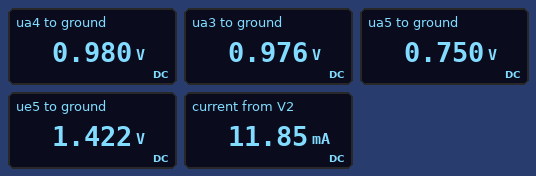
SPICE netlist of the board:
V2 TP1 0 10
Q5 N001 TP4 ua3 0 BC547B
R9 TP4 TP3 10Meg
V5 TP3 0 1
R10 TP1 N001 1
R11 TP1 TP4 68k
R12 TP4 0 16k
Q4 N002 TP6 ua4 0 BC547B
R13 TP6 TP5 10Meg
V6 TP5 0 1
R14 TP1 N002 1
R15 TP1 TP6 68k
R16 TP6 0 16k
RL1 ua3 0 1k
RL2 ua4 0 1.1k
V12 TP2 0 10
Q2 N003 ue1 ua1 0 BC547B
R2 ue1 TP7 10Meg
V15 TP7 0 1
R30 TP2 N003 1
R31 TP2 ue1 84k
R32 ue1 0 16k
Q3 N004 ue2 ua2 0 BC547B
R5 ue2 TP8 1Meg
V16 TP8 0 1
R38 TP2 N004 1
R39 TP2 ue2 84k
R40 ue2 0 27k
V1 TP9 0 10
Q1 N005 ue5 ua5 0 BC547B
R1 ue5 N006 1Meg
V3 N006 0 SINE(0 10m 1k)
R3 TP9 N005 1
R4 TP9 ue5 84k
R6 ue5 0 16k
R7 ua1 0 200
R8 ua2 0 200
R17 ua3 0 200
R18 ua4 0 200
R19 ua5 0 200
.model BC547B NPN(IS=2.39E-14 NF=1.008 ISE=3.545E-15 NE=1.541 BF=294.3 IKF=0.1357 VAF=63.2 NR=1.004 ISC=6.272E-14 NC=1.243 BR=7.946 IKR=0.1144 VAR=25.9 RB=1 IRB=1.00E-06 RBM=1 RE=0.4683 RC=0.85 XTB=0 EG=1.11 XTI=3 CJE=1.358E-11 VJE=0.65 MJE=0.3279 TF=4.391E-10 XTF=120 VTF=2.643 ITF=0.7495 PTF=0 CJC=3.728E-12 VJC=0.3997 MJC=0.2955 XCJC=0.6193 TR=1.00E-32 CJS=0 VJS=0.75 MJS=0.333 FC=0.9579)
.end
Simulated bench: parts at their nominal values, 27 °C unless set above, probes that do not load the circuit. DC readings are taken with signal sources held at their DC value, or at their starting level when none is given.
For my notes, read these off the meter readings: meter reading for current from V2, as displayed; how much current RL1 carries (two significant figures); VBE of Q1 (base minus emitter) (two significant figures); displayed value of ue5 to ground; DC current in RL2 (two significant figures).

11.85 mA
980 µA
670 mV
1.422 V
890 µA
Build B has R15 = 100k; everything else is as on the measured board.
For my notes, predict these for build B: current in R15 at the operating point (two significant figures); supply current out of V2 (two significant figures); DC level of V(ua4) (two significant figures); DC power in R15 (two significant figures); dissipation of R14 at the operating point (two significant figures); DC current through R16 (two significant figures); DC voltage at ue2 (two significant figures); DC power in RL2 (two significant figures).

88 µA
9.4 mA
570 mV
770 µW
11 µW
77 µA
2.0 V
290 µW
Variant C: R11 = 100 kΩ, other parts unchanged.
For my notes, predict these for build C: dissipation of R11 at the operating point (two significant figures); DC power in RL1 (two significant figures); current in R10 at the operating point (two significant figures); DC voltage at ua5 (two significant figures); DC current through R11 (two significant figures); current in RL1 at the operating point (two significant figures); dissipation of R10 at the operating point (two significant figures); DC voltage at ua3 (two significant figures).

770 µW
320 µW
3.4 mA
750 mV
88 µA
560 µA
11 µW
560 mV
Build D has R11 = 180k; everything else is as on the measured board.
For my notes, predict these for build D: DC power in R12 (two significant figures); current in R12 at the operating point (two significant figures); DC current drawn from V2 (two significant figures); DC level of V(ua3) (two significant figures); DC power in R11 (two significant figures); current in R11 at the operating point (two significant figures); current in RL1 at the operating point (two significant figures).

38 µW
49 µA
6.8 mA
150 mV
470 µW
51 µA
150 µA
